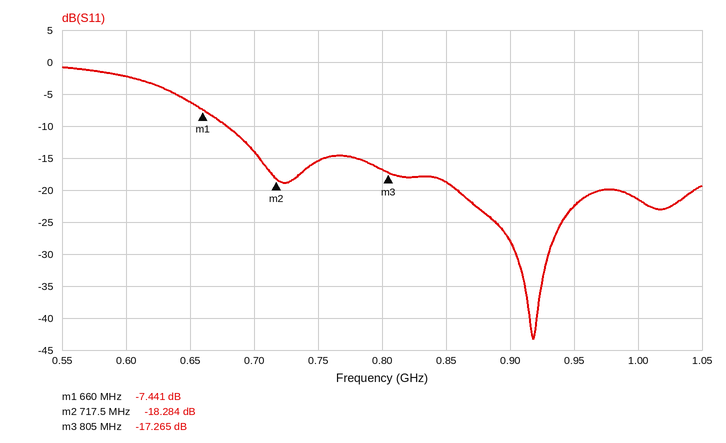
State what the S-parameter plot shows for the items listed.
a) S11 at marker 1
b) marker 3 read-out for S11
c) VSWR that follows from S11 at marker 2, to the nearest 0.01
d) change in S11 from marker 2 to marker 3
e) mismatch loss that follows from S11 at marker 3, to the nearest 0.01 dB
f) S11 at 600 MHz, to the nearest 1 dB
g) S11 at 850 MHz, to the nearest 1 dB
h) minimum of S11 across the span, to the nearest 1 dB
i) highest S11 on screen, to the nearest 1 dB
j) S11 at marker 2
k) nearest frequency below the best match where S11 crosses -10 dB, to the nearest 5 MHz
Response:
-7.441 dB
-17.265 dB
1.28
1.019 dB
0.08 dB
-2 dB
-19 dB
-43 dB
-1 dB
-18.284 dB
680 MHz
